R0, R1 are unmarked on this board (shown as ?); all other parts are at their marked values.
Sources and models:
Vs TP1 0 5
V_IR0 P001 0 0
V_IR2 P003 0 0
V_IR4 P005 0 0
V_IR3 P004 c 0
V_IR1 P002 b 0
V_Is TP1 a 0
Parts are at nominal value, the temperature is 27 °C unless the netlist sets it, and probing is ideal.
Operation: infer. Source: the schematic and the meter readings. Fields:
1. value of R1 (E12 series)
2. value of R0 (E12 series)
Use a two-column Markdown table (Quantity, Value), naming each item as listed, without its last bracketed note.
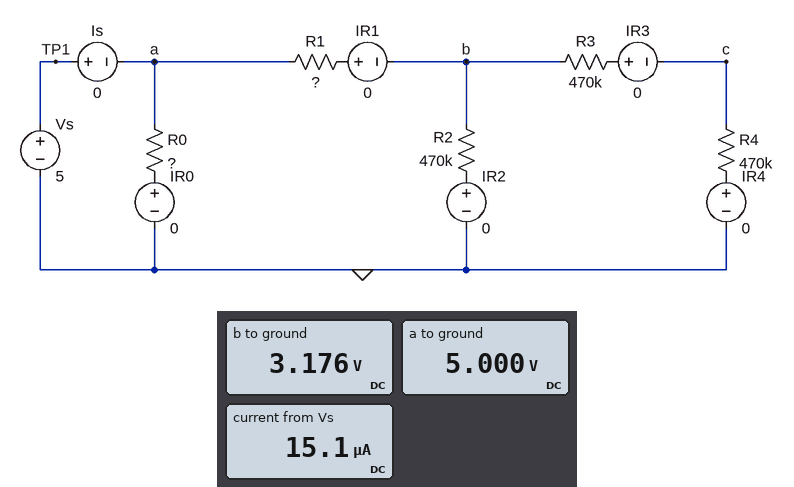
| Quantity | Value |
|---|---|
| value of R1 | 180 kΩ |
| value of R0 | 1 MΩ |
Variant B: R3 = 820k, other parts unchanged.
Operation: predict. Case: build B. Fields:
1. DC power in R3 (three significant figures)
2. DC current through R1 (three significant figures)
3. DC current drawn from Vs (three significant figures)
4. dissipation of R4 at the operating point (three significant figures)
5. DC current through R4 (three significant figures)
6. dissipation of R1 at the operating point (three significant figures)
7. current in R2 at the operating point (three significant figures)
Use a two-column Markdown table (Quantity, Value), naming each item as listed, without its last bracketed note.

| Quantity | Value |
|---|---|
| DC power in R3 | 5.31 µW |
| DC current through R1 | 9.53 µA |
| DC current drawn from Vs | 14.5 µA |
| dissipation of R4 at the operating point | 3.05 µW |
| DC current through R4 | 2.55 µA |
| dissipation of R1 at the operating point | 16.4 µW |
| current in R2 at the operating point | 6.99 µA |
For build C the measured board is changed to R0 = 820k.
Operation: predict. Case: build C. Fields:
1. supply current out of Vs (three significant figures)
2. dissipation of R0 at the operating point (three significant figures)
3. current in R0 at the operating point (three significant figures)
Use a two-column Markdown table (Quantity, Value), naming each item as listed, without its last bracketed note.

| Quantity | Value |
|---|---|
| supply current out of Vs | 16.2 µA |
| dissipation of R0 at the operating point | 30.5 µW |
| current in R0 at the operating point | 6.10 µA |
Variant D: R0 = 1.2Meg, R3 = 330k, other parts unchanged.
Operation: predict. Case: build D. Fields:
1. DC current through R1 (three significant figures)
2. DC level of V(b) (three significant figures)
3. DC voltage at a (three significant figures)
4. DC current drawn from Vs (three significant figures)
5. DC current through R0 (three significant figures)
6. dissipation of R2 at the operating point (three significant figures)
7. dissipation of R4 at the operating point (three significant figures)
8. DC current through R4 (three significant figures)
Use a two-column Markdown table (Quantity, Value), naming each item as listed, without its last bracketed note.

| Quantity | Value |
|---|---|
| DC current through R1 | 10.5 µA |
| DC level of V(b) | 3.11 V |
| DC voltage at a | 5.00 V |
| DC current drawn from Vs | 14.7 µA |
| DC current through R0 | 4.17 µA |
| dissipation of R2 at the operating point | 20.6 µW |
| dissipation of R4 at the operating point | 7.10 µW |
| DC current through R4 | 3.89 µA |
